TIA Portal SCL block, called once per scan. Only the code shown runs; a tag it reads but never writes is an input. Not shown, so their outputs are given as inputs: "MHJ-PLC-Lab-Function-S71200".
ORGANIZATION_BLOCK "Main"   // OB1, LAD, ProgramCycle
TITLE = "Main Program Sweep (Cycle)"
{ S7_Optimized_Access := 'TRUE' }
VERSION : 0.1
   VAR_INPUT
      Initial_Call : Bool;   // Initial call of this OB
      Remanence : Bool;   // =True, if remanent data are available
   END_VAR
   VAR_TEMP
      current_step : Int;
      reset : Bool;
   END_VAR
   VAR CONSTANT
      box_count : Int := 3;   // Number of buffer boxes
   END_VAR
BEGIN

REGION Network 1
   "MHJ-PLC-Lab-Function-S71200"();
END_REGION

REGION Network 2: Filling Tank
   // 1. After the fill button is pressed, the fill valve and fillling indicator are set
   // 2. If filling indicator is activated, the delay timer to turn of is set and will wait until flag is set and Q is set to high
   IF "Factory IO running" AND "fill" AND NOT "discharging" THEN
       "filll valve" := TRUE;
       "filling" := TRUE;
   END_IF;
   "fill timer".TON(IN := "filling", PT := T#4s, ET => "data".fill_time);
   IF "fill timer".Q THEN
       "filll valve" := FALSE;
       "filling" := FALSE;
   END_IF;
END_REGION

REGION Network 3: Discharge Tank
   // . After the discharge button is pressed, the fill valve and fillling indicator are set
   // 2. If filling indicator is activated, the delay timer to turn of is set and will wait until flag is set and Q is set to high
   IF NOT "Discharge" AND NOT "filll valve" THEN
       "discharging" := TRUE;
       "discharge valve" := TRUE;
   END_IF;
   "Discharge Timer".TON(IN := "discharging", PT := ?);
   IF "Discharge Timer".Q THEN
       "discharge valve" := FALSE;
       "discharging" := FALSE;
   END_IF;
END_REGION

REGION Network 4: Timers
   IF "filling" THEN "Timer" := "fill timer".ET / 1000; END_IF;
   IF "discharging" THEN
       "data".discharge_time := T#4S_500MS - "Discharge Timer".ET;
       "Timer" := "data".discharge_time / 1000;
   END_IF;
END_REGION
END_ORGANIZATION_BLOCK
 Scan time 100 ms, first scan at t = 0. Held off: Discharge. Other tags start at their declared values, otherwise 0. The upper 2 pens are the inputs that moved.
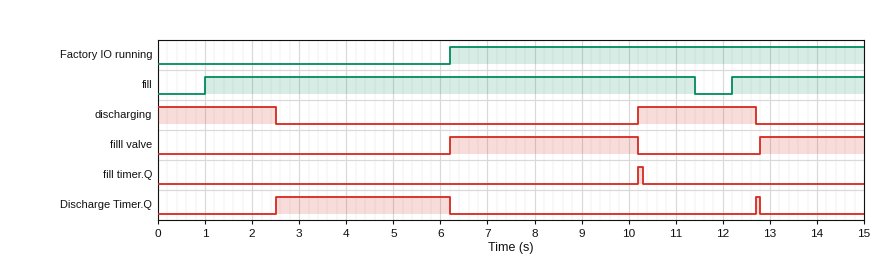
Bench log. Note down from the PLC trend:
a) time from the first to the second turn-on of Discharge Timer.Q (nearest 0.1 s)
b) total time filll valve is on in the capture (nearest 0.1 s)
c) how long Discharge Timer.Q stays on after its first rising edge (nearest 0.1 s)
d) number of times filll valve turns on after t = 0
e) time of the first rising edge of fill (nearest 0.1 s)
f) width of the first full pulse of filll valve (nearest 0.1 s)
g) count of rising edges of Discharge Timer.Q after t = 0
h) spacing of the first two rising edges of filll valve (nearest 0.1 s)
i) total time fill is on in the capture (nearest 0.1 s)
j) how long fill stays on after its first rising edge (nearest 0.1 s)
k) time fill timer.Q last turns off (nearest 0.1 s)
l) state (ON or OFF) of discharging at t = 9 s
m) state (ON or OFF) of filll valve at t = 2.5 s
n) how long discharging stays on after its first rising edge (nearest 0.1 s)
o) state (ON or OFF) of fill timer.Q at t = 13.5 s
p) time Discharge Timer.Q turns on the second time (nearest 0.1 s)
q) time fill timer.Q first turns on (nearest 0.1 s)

10.2 s
6.2 s
3.7 s
2
1.0 s
4.0 s
2
6.6 s
13.2 s
10.4 s
10.3 s
OFF
OFF
2.5 s
OFF
12.7 s
10.2 s
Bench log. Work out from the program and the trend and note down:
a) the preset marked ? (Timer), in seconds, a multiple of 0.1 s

2.5 s
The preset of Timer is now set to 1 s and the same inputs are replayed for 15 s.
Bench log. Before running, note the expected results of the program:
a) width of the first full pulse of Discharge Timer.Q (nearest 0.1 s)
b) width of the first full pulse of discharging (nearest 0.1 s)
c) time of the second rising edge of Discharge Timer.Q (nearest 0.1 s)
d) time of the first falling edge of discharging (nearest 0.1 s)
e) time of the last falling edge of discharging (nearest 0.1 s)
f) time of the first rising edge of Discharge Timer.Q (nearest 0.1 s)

5.2 s
1.0 s
11.2 s
1.0 s
11.2 s
1.0 s
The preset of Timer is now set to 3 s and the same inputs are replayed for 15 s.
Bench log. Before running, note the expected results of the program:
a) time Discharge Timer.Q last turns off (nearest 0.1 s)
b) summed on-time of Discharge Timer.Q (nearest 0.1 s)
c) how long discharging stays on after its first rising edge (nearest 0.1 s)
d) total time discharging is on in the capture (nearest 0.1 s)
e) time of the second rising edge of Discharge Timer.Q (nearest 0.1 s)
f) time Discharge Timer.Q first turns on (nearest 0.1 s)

13.3 s
3.3 s
3.0 s
6.0 s
13.2 s
3.0 s
